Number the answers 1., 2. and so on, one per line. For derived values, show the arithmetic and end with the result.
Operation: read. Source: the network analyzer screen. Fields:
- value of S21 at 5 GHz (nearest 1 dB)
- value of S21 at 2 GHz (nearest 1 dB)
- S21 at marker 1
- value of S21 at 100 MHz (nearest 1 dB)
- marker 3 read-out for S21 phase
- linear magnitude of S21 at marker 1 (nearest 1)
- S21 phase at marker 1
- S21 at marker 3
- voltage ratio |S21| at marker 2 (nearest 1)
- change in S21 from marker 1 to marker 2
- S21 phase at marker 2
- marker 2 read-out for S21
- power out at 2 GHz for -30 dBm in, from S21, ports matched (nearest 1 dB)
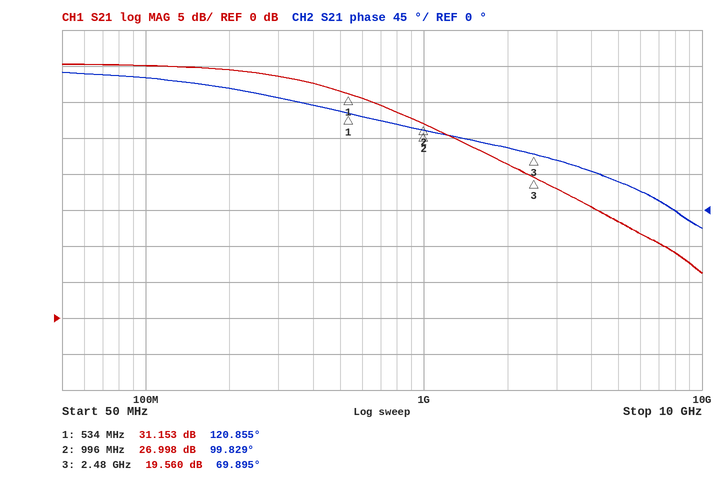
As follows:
1. 13 dB
2. 21 dB
3. 31.153 dB
4. 35 dB
5. 69.895°
6. 10^(31.153/20) ≈ 36
7. 120.855°
8. 19.560 dB
9. 10^(26.998/20) ≈ 22
10. 26.998 − (31.153) = -4.155 dB
11. 99.829°
12. 26.998 dB
13. -30 dBm + (21 dB) = -9 dBm
